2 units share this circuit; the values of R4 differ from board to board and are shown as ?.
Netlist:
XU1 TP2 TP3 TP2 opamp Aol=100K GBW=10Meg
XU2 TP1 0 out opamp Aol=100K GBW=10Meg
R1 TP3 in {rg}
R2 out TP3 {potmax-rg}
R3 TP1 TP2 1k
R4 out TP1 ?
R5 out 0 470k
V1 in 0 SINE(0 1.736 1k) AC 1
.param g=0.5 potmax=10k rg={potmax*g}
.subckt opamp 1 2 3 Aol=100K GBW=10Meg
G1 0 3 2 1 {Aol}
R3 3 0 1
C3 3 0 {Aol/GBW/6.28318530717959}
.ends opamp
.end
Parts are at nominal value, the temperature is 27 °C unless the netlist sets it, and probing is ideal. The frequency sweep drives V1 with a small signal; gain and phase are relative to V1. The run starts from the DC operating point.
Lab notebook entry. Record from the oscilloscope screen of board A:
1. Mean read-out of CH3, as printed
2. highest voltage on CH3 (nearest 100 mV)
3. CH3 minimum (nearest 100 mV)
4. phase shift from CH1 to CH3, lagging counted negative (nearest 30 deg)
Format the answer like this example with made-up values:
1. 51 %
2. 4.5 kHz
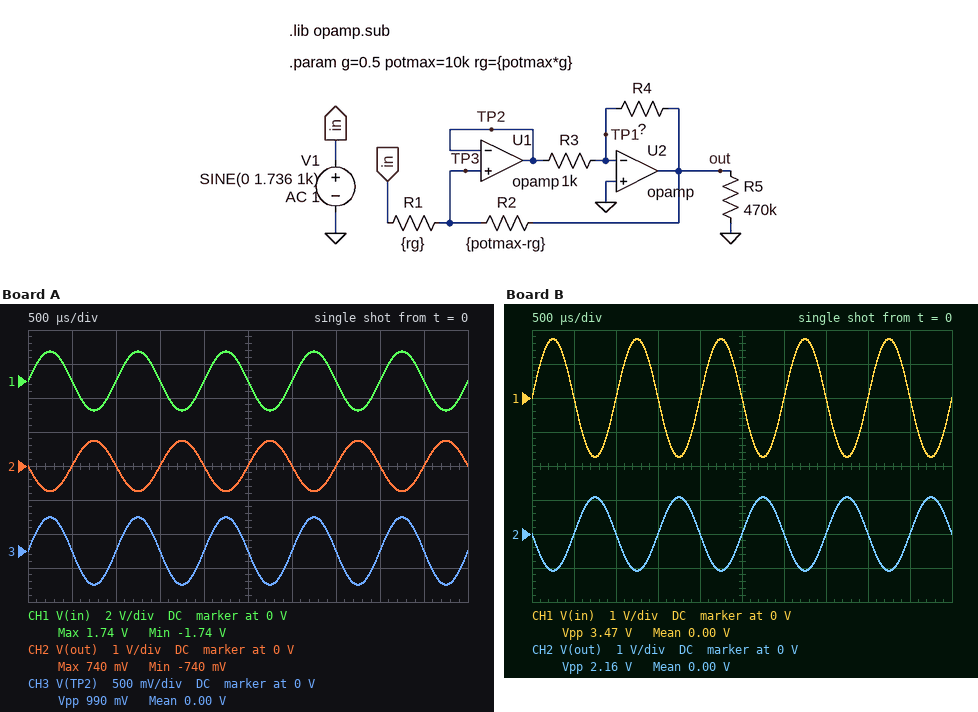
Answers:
1. 0.00 V
2. 500 mV
3. -500 mV
4. 0 deg
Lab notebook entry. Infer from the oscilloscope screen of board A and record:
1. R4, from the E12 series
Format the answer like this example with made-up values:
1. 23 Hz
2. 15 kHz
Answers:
1. 1.5 kΩ
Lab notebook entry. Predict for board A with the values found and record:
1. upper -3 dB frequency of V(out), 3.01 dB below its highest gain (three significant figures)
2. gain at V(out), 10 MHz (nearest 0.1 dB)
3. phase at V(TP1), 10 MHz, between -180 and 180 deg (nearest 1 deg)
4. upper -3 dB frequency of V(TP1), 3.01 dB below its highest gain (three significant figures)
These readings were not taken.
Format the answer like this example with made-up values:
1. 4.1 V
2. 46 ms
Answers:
1. 6.88 MHz
2. -13.6 dB
3. -12 deg
4. 17.9 MHz
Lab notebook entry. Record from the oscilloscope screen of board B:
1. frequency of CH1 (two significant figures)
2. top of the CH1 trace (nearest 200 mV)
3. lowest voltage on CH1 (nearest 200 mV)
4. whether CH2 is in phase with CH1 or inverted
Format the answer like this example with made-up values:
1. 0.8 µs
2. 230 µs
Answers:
1. 1.0 kHz
2. 1.8 V
3. -1.8 V
4. inverted
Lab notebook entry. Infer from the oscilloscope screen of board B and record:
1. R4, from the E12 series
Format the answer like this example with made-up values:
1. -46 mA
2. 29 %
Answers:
1. 3.3 kΩ
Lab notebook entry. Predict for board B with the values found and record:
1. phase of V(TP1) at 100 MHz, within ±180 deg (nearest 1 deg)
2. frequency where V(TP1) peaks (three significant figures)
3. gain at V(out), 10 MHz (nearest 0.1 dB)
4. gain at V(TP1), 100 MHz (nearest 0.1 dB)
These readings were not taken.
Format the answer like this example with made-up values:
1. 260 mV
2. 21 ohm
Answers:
1. -83 deg
2. 7.85 MHz
3. -10.5 dB
4. -28.3 dB
